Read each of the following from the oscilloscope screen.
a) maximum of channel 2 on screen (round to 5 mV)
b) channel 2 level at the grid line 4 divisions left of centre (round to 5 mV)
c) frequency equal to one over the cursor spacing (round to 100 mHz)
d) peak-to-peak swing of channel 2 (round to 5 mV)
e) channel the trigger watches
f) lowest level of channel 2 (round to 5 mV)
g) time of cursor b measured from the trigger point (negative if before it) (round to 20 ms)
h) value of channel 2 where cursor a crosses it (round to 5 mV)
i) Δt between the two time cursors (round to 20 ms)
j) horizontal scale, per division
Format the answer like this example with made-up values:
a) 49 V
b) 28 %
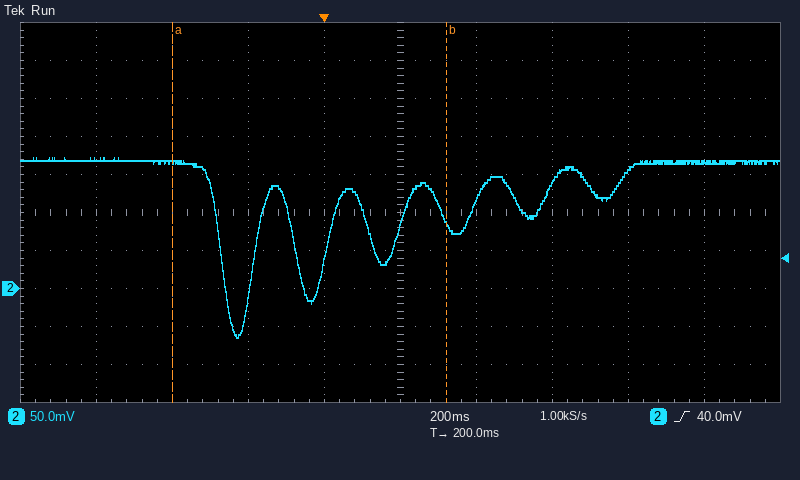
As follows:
a) 170 mV
b) 170 mV
c) 1.4 Hz
d) 235 mV
e) channel 2
f) -65 mV
g) +320 ms
h) 165 mV
i) 720 ms
j) 200 ms
